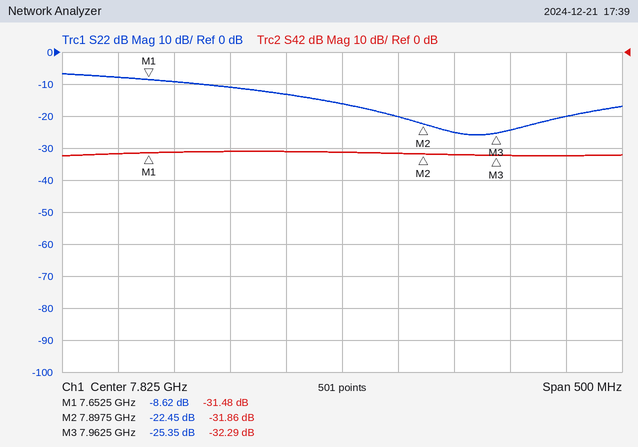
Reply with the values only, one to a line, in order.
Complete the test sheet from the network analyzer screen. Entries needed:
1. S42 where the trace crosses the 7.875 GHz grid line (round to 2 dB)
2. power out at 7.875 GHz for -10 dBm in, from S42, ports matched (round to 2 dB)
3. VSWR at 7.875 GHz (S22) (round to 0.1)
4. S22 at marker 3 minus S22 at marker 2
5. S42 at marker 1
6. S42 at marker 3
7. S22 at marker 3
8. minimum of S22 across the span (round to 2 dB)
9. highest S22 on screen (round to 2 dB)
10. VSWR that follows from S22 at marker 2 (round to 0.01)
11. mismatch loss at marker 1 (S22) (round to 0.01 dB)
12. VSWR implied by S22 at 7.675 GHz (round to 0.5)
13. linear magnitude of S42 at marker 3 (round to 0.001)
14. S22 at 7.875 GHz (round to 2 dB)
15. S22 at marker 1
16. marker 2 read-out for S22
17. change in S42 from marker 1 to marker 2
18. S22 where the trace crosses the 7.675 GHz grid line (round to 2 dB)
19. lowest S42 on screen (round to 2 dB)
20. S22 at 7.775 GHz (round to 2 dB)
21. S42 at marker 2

-32 dB
-42 dBm
1.2
-2.90 dB
-31.48 dB
-32.29 dB
-25.35 dB
-26 dB
-6 dB
1.16
0.64 dB
2.0
0.024
-20 dB
-8.62 dB
-22.45 dB
-0.38 dB
-10 dB
-32 dB
-14 dB
-31.86 dB
